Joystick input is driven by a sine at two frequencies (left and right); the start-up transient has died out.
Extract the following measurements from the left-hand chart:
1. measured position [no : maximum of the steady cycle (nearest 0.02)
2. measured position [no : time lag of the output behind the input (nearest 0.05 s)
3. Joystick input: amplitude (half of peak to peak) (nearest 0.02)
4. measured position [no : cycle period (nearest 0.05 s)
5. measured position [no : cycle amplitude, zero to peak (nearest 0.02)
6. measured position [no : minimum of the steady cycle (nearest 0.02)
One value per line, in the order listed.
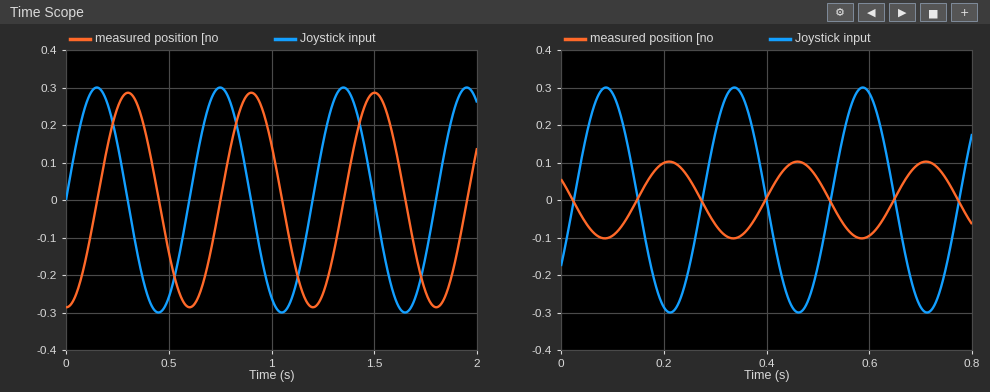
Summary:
0.28
0.15 s
0.30
0.60 s
0.28
-0.28
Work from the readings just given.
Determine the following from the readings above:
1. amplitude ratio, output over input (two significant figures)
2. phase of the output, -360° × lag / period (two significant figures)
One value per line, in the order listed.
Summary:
0.93
-90°
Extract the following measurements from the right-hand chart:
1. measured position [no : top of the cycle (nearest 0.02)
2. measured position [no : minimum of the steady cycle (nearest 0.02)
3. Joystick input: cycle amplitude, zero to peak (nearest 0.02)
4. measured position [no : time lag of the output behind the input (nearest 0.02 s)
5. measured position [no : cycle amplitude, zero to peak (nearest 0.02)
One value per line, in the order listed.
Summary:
0.10
-0.10
0.30
0.12 s
0.10
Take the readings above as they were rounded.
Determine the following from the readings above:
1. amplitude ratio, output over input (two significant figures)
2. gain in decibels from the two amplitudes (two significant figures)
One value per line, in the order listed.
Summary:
0.33
-9.5 dB
